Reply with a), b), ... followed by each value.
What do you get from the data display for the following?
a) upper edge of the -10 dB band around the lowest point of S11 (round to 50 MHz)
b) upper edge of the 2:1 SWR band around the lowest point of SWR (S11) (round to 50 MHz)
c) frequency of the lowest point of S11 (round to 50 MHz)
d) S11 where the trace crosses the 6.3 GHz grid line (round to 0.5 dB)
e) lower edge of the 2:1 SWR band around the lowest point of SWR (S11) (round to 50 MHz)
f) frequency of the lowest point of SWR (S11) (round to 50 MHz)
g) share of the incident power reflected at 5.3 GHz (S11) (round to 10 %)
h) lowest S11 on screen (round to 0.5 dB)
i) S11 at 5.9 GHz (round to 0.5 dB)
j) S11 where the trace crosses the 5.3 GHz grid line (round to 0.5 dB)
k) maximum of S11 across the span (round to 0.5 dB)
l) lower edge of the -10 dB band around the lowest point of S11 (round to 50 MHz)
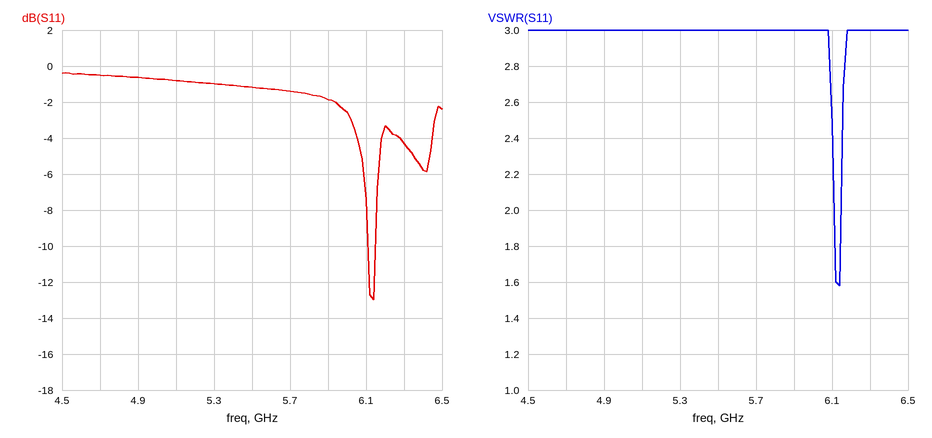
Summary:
a) 6.15 GHz
b) 6.15 GHz
c) 6.15 GHz
d) -4.5 dB
e) 6.10 GHz
f) 6.15 GHz
g) 80 %
h) -13.0 dB
i) -2.0 dB
j) -1.0 dB
k) -0.5 dB
l) 6.10 GHz
